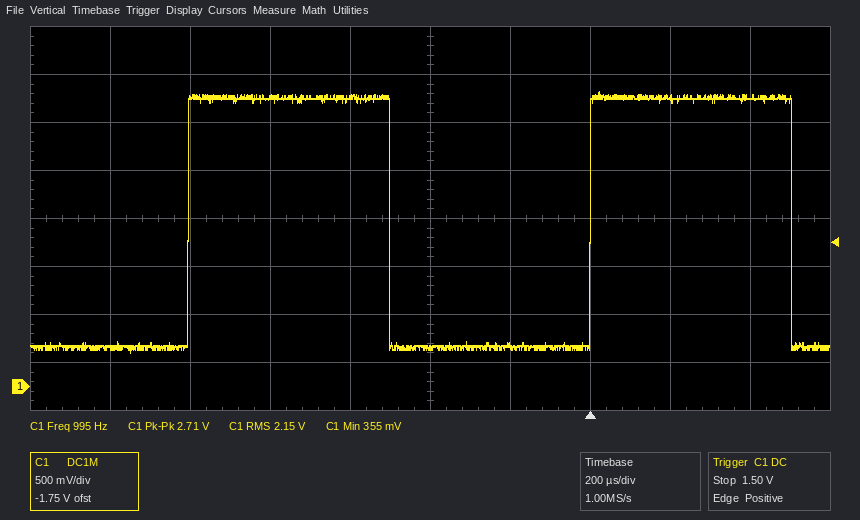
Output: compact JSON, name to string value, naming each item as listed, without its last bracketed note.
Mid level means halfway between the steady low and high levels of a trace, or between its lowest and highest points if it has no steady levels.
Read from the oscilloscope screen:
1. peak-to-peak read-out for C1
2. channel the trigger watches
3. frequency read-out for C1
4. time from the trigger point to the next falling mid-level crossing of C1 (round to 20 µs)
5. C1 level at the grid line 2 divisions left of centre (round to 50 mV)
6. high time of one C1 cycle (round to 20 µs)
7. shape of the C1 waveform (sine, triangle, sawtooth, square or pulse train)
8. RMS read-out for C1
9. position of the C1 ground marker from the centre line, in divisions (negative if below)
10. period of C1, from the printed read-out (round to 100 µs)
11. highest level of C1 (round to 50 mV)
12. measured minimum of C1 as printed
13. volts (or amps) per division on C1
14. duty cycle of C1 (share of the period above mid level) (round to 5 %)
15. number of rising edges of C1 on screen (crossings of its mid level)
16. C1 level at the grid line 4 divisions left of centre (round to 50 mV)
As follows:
{"peak-to-peak read-out for C1": "2.71 V", "channel the trigger watches": "C1", "frequency read-out for C1": "995 Hz", "time from the trigger point to the next falling mid-level crossing of C1": "500 µs", "C1 level at the grid line 2 divisions left of centre": "3.00 V", "high time of one C1 cycle": "500 µs", "shape of the C1 waveform": "square", "RMS read-out for C1": "2.15 V", "position of the C1 ground marker from the centre line, in divisions": "-3.5 div", "period of C1, from the printed read-out": "1.0 ms", "highest level of C1": "3.05 V", "measured minimum of C1 as printed": "355 mV", "volts (or amps) per division on C1": "500 mV", "duty cycle of C1 (share of the period above mid level)": "50 %", "number of rising edges of C1 on screen": "2", "C1 level at the grid line 4 divisions left of centre": "400 mV"}
